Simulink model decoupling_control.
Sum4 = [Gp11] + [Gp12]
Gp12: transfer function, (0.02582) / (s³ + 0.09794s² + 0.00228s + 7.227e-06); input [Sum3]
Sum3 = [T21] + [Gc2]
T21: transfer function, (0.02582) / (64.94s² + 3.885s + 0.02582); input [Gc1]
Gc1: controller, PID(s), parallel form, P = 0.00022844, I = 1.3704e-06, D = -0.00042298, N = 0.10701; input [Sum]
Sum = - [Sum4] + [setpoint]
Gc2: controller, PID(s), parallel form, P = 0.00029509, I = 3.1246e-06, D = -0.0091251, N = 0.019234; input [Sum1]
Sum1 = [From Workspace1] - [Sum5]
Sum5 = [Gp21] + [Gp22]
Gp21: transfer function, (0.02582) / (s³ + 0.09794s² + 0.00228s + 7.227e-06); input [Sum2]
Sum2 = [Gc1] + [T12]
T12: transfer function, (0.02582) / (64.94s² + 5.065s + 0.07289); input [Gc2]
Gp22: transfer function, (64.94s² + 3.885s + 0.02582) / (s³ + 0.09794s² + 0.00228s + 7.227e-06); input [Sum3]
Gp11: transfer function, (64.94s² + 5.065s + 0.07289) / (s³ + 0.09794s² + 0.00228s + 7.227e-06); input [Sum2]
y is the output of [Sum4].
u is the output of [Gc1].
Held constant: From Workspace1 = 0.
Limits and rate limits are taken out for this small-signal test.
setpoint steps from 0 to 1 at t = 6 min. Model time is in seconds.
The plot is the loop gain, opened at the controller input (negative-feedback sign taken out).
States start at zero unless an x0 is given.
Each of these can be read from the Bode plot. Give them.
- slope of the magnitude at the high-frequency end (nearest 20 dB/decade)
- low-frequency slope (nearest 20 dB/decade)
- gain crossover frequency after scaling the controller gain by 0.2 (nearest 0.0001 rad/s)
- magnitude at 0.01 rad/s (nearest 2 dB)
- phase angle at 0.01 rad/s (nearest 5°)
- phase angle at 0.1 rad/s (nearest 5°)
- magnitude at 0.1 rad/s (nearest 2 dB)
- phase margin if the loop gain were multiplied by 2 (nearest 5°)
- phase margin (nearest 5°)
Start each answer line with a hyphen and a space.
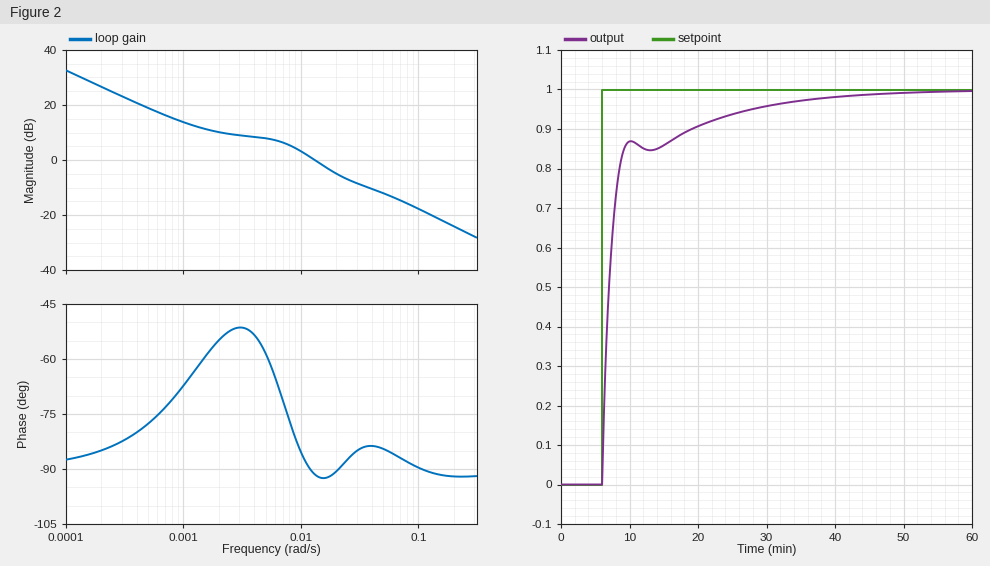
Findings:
- -20 dB/decade
- -20 dB/decade
- 0.0010 rad/s
- 4 dB
- -85°
- -90°
- -18 dB
- 90°
- 90°
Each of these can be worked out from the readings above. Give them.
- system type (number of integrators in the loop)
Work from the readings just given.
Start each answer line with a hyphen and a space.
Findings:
- 1
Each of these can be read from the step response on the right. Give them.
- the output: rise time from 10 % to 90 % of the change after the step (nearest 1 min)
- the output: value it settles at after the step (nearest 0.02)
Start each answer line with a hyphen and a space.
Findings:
- 13 min
- 1.00
